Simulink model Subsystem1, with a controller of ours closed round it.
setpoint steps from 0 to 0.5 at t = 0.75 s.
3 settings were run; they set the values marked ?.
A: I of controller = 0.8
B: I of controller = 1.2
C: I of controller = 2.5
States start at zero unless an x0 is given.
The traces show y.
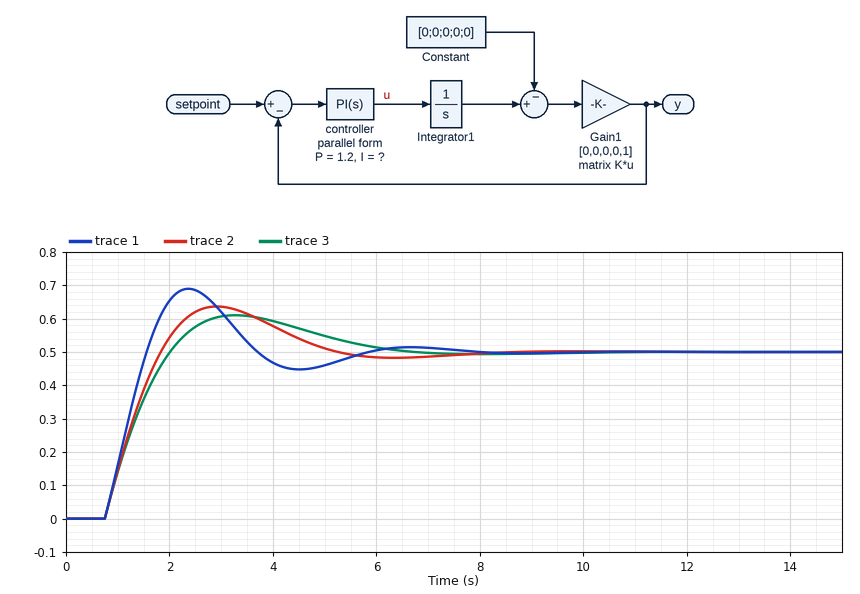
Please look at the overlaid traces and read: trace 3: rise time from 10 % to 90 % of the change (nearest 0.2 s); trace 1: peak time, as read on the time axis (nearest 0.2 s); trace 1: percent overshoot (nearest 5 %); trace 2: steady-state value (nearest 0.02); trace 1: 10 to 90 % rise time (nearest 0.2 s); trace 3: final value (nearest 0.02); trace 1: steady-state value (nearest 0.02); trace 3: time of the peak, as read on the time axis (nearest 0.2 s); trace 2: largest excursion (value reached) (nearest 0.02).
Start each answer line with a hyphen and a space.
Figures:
- 1.0 s
- 2.4 s
- 40 %
- 0.50
- 0.6 s
- 0.50
- 0.50
- 3.2 s
- 0.64
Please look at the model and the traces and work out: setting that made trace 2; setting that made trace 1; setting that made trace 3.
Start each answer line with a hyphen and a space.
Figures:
- B
- C
- A
